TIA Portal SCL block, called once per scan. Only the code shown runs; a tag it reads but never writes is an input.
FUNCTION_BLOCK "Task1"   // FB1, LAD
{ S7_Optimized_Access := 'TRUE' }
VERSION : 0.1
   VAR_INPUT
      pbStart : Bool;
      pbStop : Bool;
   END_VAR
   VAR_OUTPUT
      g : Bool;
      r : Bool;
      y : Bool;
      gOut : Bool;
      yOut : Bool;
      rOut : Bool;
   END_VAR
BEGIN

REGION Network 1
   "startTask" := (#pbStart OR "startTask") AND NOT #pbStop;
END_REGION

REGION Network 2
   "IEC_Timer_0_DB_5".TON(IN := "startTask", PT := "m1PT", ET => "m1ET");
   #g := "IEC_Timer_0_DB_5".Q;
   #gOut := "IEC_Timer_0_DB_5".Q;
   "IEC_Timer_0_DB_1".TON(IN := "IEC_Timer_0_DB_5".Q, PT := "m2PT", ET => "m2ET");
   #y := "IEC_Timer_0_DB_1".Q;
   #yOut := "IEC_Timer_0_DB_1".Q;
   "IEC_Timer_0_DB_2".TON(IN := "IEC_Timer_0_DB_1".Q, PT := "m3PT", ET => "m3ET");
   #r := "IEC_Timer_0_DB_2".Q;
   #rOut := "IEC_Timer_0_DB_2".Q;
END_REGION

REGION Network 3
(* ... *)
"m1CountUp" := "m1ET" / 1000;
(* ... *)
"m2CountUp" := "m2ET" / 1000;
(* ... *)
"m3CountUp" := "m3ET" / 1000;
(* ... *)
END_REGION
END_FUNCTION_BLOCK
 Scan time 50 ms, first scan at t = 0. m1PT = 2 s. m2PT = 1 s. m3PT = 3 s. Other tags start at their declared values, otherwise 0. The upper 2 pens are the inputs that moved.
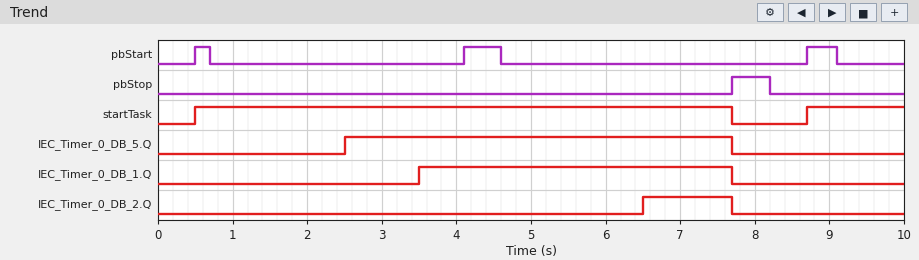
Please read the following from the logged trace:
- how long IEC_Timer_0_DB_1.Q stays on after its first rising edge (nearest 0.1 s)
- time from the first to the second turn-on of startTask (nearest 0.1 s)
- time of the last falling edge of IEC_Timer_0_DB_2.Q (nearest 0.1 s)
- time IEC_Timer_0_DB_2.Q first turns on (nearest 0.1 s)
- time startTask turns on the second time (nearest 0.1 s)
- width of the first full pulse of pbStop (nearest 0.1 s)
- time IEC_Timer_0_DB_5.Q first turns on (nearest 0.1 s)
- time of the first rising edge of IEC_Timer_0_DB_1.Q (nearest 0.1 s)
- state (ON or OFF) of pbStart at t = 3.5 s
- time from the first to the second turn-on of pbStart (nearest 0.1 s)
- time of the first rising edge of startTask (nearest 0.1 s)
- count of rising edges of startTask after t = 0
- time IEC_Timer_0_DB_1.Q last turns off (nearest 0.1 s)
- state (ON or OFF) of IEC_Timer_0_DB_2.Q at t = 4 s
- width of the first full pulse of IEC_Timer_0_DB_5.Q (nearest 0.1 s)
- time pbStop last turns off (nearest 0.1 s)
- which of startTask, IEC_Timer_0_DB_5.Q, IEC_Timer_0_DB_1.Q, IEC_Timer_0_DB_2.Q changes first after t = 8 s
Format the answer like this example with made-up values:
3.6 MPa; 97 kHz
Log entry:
4.2 s; 8.2 s; 7.7 s; 6.5 s; 8.7 s; 0.5 s; 2.5 s; 3.5 s; OFF; 3.6 s; 0.5 s; 2; 7.7 s; OFF; 5.2 s; 8.2 s; startTask
